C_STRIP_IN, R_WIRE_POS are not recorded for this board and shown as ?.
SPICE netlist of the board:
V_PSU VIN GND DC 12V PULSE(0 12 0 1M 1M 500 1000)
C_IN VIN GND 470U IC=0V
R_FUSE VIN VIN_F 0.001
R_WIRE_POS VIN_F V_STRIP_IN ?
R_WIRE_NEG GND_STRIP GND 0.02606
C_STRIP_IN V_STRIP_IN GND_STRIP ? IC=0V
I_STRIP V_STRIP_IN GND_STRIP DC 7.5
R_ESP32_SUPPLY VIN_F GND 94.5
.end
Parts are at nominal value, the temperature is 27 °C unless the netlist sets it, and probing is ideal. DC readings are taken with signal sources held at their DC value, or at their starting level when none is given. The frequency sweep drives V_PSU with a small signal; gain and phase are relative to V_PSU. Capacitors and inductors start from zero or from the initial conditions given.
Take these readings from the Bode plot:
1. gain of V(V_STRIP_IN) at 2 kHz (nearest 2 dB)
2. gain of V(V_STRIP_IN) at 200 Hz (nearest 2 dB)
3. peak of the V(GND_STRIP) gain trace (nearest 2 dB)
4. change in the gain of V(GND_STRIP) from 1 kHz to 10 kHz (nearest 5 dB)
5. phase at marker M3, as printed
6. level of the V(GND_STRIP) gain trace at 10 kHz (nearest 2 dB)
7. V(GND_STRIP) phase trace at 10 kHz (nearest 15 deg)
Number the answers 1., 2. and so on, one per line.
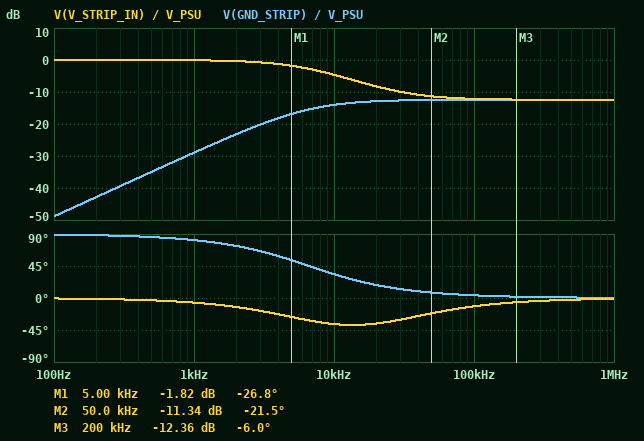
1. 0 dB
2. 0 dB
3. -12 dB
4. 15 dB
5. -6.0 deg
6. -14 dB
7. 30 deg
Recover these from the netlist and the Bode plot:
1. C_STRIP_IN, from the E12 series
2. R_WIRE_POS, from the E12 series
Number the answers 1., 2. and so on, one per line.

1. 220 µF
2. 0.082 Ω
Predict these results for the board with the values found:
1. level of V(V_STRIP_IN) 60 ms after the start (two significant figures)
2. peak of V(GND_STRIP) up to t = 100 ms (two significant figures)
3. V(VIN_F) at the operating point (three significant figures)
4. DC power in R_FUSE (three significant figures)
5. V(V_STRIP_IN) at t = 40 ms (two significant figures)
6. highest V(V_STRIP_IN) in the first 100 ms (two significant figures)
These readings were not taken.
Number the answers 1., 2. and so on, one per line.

1. 11 V
2. 260 mV
3. 12.0 V
4. 58.2 mW
5. 11 V
6. 11 V
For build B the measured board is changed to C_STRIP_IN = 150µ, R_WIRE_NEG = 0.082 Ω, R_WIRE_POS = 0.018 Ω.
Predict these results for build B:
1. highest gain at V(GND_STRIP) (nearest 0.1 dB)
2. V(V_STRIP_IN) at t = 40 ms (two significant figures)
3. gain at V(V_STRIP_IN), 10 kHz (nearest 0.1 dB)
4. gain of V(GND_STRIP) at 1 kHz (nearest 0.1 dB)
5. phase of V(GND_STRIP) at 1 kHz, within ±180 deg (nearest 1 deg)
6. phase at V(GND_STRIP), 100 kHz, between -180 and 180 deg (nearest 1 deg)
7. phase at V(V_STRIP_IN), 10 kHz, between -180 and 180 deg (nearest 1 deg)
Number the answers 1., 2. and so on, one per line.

1. -1.8 dB
2. 12 V
3. -0.8 dB
4. -22.3 dB
5. 85 deg
6. 6 deg
7. -6 deg
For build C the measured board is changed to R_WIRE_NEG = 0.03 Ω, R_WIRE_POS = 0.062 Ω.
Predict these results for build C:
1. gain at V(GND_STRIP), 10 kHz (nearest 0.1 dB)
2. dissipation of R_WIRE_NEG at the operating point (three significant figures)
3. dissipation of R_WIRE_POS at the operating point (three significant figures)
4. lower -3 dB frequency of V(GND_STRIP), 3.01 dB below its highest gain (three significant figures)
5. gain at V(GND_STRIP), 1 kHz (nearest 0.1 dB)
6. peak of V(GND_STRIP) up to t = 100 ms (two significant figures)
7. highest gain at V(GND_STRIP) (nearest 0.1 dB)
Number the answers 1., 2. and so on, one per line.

1. -11.9 dB
2. 1.69 W
3. 3.49 W
4. 7.78 kHz
5. -27.7 dB
6. 300 mV
7. -9.8 dB
